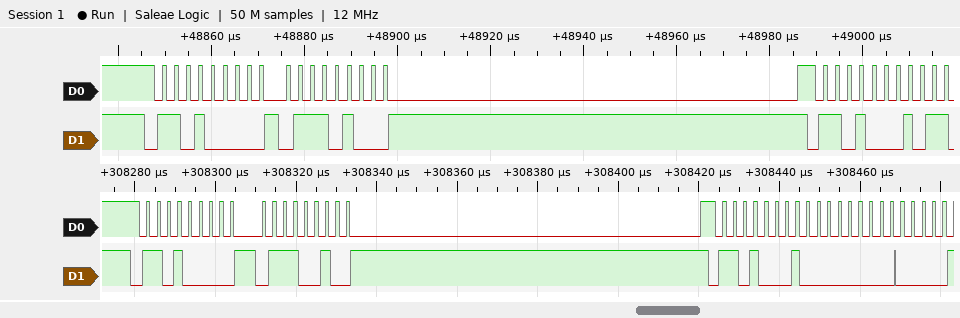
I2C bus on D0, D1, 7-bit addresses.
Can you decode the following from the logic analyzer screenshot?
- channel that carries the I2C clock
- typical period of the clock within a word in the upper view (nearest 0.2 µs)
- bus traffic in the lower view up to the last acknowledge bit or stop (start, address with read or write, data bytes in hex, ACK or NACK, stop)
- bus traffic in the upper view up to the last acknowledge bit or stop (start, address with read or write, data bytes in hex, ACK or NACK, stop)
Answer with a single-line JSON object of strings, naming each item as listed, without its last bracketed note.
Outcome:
{"channel that carries the I2C clock": "D0", "typical period of the clock within a word in the upper view": "2.6 µs", "bus traffic in the lower view up to the last acknowledge bit or stop": "start, address 68 write ACK, 72 ACK, repeated start, address 68 read ACK, 00 ACK", "bus traffic in the upper view up to the last acknowledge bit or stop": "start, address 68 write ACK, 74 ACK, repeated start, address 68 read ACK"}
